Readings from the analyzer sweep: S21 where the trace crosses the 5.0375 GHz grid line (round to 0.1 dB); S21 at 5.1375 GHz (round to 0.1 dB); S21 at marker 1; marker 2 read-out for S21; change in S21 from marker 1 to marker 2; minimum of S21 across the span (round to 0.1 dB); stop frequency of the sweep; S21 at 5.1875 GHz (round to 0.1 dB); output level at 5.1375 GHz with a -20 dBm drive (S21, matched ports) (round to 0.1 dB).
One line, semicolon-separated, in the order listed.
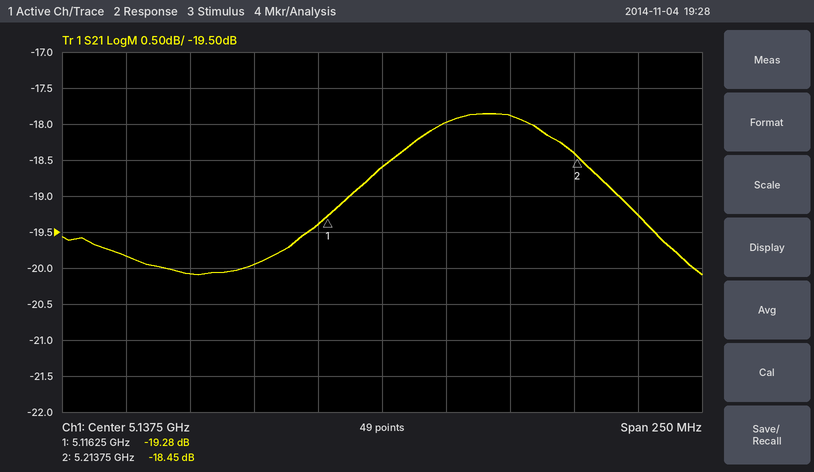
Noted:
-19.8 dB; -18.6 dB; -19.28 dB; -18.45 dB; 0.83 dB; -20.1 dB; 5.2625 GHz; -17.9 dB; -38.6 dBm
